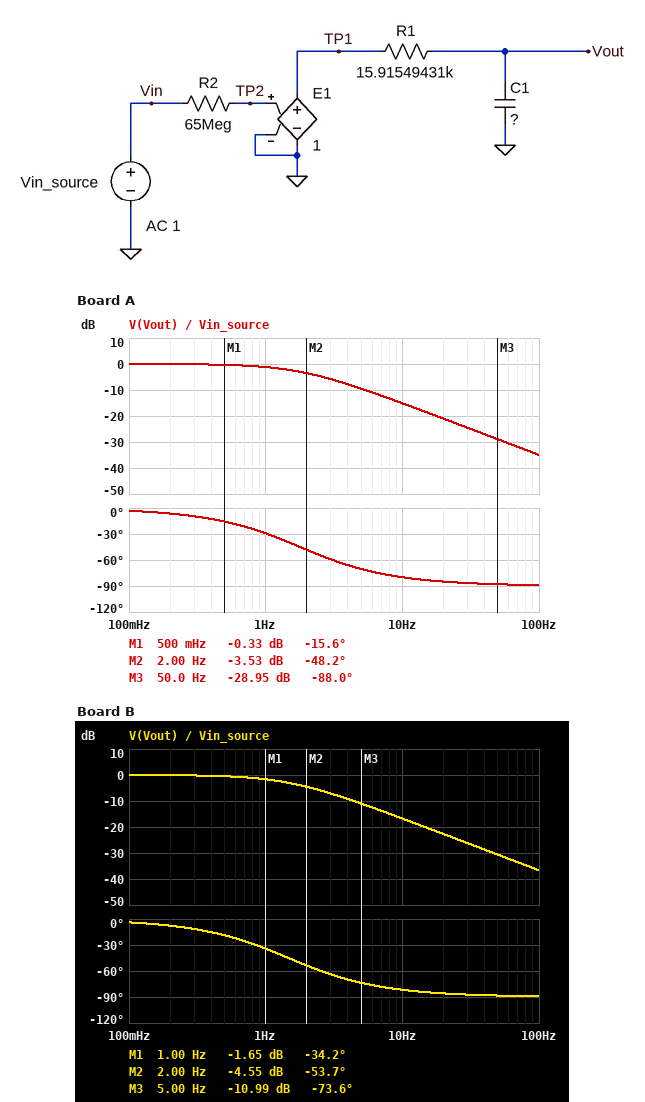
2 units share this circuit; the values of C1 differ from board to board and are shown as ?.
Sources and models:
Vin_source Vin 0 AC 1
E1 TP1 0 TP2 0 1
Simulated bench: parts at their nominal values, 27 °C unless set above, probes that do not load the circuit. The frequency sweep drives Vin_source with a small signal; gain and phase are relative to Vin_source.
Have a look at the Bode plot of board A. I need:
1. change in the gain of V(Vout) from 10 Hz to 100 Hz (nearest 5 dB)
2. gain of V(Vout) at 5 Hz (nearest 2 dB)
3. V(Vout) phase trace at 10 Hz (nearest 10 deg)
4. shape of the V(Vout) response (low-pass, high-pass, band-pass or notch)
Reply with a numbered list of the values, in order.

1. -20 dB
2. -10 dB
3. -80 deg
4. low-pass
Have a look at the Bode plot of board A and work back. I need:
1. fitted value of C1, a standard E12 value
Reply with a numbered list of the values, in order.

1. 5.6 µF
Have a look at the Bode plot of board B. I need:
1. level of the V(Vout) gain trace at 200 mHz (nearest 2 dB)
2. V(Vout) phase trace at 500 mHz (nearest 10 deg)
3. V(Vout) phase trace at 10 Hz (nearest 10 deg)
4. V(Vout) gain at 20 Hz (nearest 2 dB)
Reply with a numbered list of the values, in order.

1. 0 dB
2. -20 deg
3. -80 deg
4. -22 dB
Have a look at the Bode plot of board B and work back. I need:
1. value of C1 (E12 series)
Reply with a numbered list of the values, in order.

1. 6.8 µF
